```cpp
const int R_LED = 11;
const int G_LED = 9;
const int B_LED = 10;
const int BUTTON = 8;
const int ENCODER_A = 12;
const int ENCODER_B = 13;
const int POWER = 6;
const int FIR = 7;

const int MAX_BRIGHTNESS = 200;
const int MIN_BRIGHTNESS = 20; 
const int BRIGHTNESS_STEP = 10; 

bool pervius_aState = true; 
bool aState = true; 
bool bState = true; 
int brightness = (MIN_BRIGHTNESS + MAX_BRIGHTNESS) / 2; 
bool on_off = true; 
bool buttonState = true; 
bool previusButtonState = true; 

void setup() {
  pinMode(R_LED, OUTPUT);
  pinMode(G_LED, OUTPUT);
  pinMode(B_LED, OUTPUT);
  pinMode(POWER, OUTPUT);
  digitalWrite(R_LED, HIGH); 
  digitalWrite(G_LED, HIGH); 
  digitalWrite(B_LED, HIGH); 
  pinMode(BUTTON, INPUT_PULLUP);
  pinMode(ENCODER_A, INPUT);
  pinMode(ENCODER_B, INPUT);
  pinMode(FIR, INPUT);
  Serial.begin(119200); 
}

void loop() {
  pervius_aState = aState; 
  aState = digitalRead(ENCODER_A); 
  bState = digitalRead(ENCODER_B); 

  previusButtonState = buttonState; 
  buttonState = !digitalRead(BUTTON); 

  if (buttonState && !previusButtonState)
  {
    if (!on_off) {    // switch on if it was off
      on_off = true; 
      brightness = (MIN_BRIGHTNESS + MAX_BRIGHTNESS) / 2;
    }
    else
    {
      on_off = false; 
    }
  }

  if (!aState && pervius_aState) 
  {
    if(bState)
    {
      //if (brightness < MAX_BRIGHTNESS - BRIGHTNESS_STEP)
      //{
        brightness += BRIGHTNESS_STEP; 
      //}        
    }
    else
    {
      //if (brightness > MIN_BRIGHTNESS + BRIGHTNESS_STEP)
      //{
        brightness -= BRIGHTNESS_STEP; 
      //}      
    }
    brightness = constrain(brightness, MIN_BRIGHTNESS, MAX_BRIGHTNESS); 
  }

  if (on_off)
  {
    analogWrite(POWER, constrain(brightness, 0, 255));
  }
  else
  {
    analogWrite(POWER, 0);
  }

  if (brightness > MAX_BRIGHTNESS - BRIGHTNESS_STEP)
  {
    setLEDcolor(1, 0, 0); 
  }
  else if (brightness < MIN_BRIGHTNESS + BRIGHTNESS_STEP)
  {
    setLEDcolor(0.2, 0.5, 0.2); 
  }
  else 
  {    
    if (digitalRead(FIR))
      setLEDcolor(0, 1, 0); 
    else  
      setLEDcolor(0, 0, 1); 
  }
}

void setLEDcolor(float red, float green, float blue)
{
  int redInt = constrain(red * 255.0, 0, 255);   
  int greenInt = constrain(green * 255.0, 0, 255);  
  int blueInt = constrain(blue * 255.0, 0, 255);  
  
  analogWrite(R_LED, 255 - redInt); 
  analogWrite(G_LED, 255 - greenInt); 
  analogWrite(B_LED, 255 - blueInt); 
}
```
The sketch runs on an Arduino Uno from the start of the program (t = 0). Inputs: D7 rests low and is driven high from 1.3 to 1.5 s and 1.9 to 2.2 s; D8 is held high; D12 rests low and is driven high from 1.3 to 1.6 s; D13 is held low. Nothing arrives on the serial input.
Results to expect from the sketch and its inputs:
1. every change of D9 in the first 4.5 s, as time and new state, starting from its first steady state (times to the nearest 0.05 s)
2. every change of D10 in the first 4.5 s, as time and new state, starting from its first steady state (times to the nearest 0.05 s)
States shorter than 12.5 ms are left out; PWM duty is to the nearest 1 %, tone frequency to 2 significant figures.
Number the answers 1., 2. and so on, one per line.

1. 0 s high; 1.3 s low; 1.5 s high; 1.9 s low; 2.2 s high
2. 0 s low; 1.3 s high; 1.5 s low; 1.9 s high; 2.2 s low
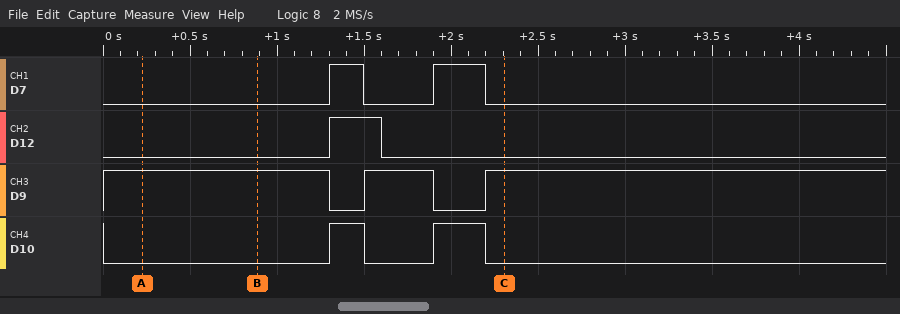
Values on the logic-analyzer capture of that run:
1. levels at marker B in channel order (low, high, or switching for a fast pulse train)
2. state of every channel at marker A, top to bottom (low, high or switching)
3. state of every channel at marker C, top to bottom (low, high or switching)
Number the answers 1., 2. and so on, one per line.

1. D7 low, D12 low, D9 high, D10 low
2. D7 low, D12 low, D9 high, D10 low
3. D7 low, D12 low, D9 high, D10 low
